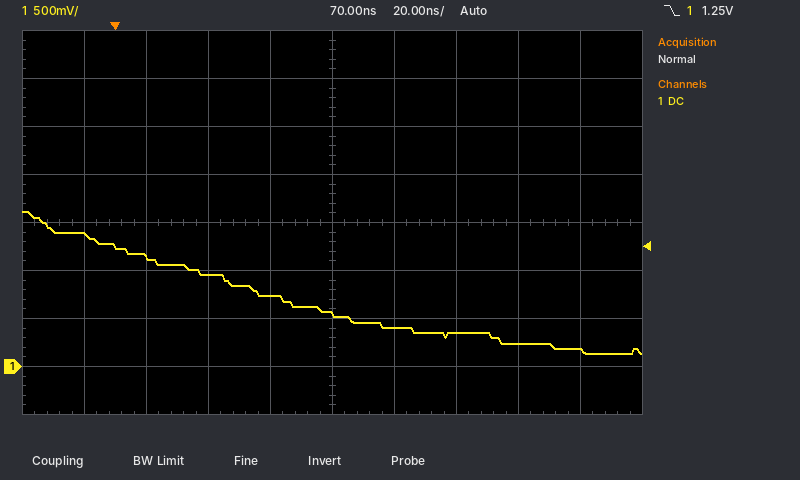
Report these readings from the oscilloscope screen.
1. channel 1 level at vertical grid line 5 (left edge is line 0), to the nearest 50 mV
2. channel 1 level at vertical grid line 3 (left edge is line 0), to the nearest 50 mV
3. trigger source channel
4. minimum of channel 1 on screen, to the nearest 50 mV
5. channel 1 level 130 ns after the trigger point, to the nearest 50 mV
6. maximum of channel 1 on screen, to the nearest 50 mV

550 mV
950 mV
channel 1
150 mV
250 mV
1.60 V
